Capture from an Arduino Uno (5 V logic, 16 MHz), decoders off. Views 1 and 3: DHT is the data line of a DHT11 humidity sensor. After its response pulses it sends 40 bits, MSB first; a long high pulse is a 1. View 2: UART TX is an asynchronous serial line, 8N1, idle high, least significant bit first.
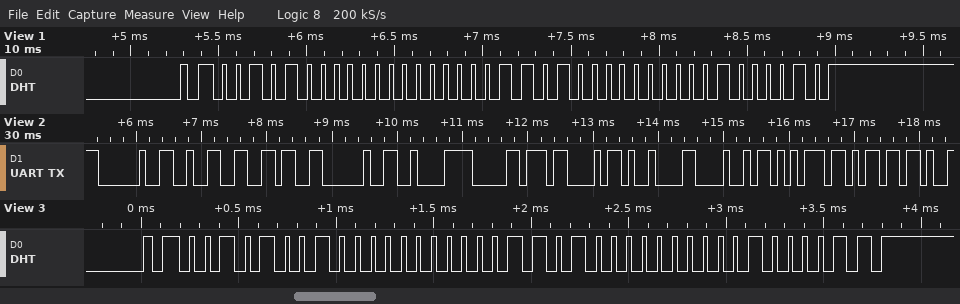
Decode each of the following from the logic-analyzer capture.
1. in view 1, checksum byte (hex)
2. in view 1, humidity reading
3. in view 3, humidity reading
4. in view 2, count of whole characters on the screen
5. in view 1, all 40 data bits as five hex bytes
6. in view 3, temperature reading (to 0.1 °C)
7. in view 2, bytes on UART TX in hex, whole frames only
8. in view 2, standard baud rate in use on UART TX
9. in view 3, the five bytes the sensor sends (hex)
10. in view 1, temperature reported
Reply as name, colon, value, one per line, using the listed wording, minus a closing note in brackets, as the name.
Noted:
in view 1, checksum byte: 0x42
in view 1, humidity reading: 40 %
in view 3, humidity reading: 41 %
in view 2, count of whole characters on the screen: 11
in view 1, all 40 data bits as five hex bytes: 28 00 1A 00 42
in view 3, temperature reading: 26.0 °C
in view 2, bytes on UART TX in hex, whole frames only: 20 32 36 20 C2 B0 43 09 48 75 6D
in view 2, standard baud rate in use on UART TX: 9600 baud
in view 3, the five bytes the sensor sends: 29 00 1A 00 43
in view 1, temperature reported: 26.0 °C
